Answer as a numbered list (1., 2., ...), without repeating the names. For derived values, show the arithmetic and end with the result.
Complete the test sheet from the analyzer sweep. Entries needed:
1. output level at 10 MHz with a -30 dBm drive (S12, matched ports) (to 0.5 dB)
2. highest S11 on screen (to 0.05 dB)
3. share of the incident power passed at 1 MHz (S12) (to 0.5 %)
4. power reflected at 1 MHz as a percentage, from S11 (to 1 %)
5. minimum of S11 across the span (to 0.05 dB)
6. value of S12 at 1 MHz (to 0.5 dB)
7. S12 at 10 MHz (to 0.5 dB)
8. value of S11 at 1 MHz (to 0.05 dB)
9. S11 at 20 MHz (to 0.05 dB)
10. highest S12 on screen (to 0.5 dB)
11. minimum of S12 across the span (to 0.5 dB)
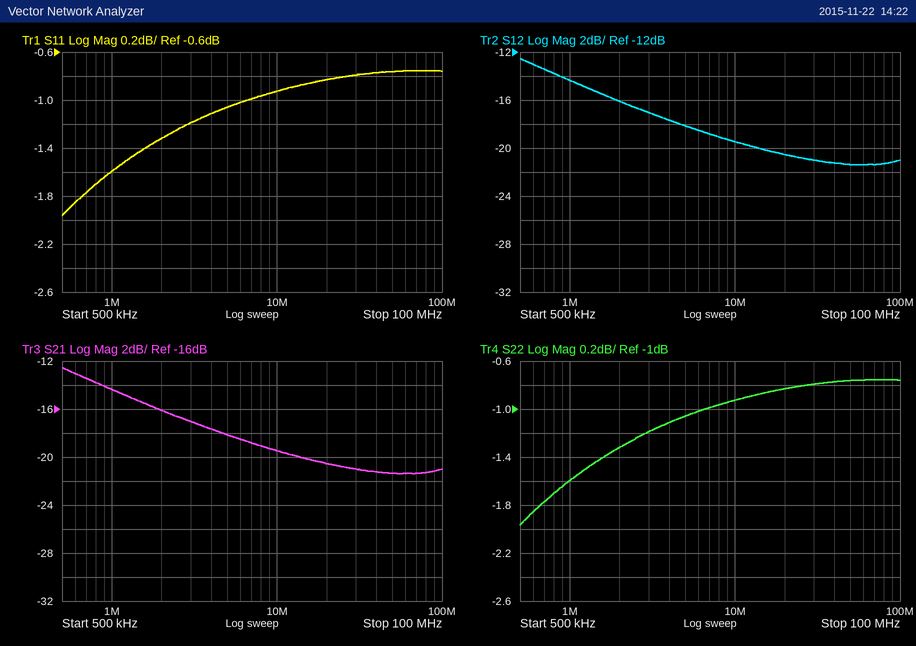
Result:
1. -30 dBm + (-19.5 dB) = -49.5 dBm
2. -0.75 dB
3. 10^(-14.5/10) ≈ 3.5 %
4. 10^(-1.6/10) ≈ 69 %
5. -1.95 dB
6. -14.5 dB
7. -19.5 dB
8. -1.60 dB
9. -0.85 dB
10. -12.5 dB
11. -21.5 dB
